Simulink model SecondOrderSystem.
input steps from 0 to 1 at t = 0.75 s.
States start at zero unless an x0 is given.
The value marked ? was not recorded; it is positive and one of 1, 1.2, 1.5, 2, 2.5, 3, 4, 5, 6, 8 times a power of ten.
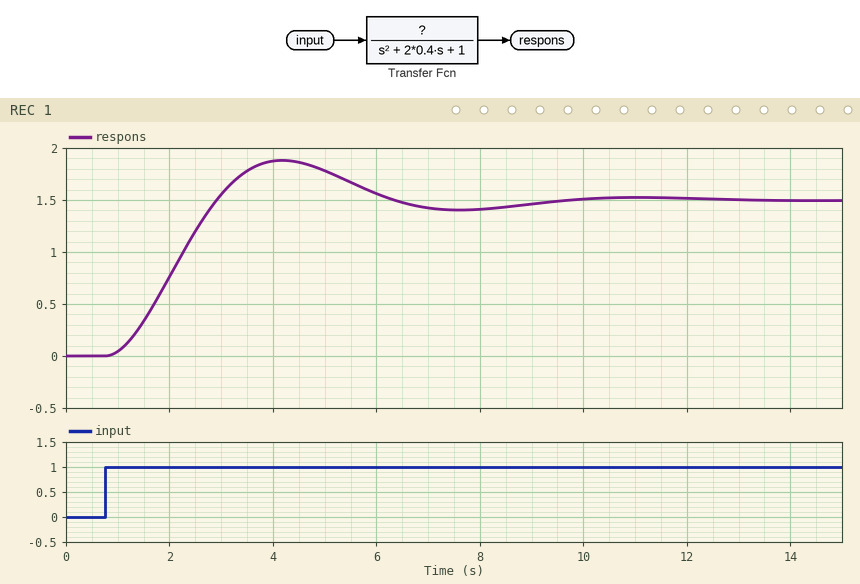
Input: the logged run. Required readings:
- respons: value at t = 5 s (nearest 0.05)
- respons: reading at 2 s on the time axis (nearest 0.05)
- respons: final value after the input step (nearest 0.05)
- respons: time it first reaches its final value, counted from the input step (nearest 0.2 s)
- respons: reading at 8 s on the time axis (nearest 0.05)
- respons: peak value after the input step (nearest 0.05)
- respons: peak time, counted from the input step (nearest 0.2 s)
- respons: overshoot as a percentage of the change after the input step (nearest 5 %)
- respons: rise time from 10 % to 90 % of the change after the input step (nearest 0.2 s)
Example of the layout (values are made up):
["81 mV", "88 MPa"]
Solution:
["1.80", "0.75", "1.50", "2.2 s", "1.40", "1.90", "3.4 s", "25 %", "1.4 s"]
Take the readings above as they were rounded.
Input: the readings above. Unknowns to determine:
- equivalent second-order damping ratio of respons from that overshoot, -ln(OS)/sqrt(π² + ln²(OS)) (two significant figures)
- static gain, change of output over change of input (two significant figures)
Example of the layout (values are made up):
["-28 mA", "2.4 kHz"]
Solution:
["0.40", "1.5"]
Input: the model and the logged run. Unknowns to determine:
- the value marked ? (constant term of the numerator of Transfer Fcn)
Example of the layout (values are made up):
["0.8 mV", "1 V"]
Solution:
["1.5"]
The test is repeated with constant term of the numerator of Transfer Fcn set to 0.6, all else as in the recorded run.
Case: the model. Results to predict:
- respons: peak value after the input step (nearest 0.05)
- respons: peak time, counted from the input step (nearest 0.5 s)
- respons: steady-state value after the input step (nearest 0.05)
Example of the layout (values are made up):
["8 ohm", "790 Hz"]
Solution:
["0.75", "3.5 s", "0.60"]
